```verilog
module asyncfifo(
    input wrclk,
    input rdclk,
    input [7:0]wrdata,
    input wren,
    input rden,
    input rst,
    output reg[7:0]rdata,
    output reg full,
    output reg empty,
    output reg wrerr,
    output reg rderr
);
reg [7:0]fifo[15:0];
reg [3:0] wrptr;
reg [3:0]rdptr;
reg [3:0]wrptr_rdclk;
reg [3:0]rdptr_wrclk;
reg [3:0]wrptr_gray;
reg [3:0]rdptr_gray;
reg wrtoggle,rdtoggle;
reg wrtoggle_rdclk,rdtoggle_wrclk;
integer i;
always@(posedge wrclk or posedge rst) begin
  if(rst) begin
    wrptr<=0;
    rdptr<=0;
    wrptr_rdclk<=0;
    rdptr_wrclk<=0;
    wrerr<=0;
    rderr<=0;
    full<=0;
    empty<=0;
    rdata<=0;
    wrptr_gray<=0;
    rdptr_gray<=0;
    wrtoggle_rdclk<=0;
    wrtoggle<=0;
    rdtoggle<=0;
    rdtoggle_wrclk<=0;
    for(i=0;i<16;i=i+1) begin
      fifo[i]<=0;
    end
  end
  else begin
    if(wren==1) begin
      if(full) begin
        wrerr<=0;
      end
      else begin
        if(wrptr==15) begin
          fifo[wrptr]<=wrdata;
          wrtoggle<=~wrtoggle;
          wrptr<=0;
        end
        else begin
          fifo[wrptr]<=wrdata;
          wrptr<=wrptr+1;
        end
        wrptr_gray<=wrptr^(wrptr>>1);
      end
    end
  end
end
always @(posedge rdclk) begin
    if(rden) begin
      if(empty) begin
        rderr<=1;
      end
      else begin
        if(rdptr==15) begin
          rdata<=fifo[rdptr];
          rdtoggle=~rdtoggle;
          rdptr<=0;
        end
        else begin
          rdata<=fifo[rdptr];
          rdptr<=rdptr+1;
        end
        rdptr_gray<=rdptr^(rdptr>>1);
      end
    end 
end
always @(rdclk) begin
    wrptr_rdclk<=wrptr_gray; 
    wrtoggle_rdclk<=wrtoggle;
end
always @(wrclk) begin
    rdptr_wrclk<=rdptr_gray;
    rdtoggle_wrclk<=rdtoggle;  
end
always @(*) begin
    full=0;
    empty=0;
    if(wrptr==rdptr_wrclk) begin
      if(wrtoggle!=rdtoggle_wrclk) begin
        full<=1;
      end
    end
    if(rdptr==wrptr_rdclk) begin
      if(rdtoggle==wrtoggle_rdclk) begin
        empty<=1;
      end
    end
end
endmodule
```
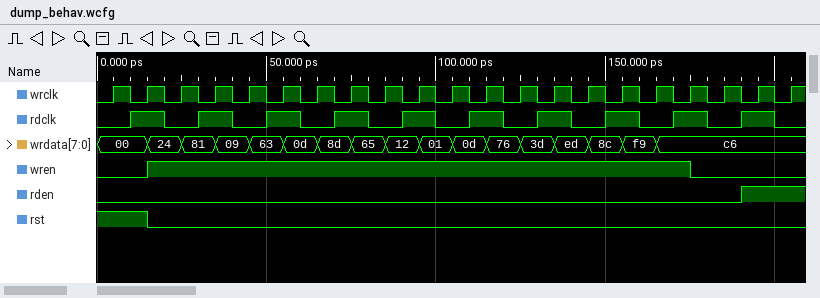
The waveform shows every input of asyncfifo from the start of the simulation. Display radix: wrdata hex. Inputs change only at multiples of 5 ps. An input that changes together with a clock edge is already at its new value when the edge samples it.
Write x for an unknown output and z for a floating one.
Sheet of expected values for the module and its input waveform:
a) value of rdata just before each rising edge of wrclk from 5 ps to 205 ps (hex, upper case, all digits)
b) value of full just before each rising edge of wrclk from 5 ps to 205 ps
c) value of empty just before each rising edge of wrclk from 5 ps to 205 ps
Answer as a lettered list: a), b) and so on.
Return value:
a) 00, 00, 00, 00, 00, 00, 00, 00, 00, 00, 00, 00, 00, 00, 00, 00, 00, 00, 00, 24, 24
b) 0 0 0 0 0 0 0 0 0 0 0 0 0 0 0 0 0 1 1 1 1
c) 1 0 1 0 0 0 0 0 0 0 0 0 0 0 0 0 0 0 0 0 0
